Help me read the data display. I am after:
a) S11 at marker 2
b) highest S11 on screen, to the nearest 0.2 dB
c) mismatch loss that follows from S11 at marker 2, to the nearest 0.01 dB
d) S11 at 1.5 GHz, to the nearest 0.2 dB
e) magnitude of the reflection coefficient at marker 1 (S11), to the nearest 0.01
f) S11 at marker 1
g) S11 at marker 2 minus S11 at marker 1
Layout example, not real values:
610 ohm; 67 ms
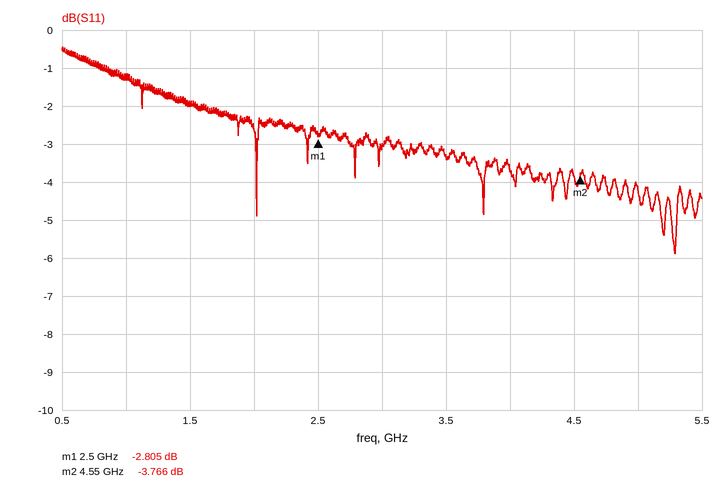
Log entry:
-3.766 dB; -0.4 dB; 2.37 dB; -2.0 dB; 0.72; -2.805 dB; -0.961 dB
